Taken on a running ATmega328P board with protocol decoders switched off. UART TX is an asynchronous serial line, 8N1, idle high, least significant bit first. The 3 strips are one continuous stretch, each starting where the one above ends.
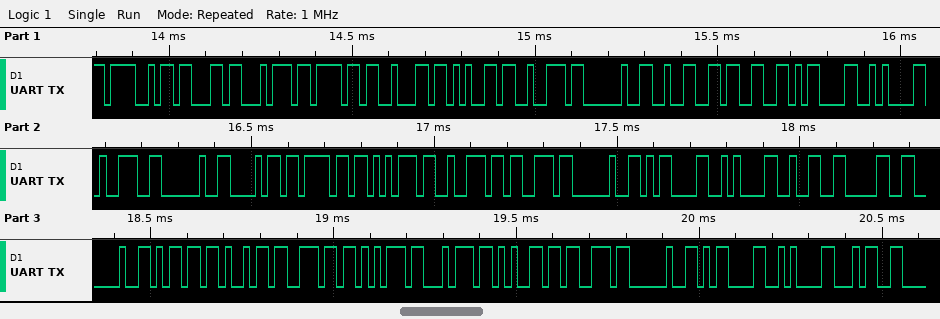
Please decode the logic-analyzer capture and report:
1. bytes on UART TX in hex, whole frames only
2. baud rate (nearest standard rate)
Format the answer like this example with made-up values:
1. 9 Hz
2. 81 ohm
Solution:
1. 0x4F 0x63 0x74 0x6F 0x62 0x65 0x72 0x20 0x32 0x33 0x0D 0x0A 0x39 0x20 0x68 0x6F 0x75 0x72 0x73 0x20 0x0D 0x0A 0x32 0x30 0x20 0x6D 0x69 0x6E 0x75 0x74 0x65 0x73 0x20 0x0D 0x0A 0x34
2. 57600 baud
